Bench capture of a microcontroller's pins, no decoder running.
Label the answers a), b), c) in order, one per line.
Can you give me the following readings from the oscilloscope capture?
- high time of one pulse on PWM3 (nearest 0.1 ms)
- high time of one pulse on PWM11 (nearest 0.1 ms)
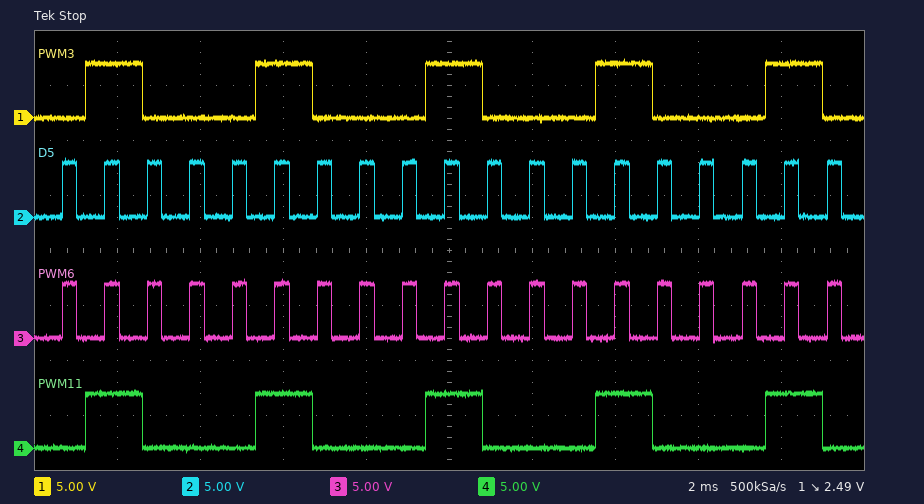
a) 1.4 ms
b) 1.4 ms
